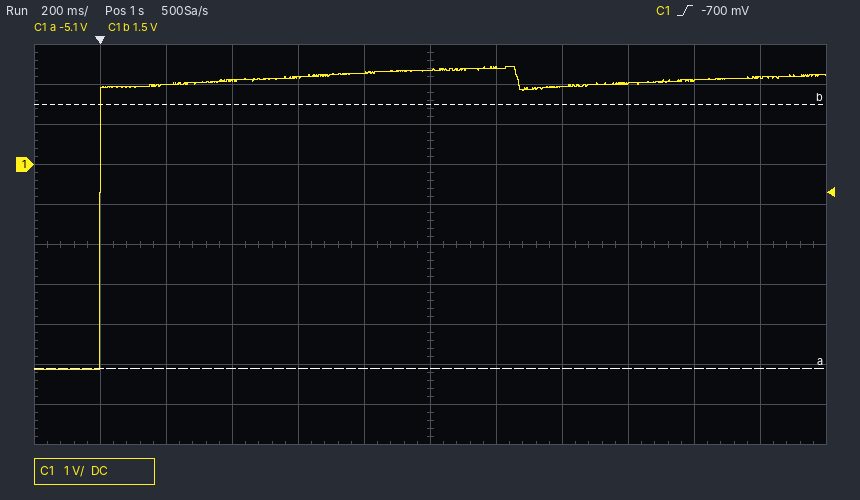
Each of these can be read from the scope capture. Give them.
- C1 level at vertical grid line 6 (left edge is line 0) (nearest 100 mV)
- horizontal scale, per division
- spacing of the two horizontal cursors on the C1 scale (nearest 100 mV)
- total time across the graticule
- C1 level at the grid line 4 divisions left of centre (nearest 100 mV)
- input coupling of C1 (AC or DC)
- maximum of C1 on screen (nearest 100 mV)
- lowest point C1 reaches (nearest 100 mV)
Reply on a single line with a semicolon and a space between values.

2.4 V; 200 ms; 6.6 V; 2.4 s; 2.0 V; DC; 2.4 V; -5.1 V
